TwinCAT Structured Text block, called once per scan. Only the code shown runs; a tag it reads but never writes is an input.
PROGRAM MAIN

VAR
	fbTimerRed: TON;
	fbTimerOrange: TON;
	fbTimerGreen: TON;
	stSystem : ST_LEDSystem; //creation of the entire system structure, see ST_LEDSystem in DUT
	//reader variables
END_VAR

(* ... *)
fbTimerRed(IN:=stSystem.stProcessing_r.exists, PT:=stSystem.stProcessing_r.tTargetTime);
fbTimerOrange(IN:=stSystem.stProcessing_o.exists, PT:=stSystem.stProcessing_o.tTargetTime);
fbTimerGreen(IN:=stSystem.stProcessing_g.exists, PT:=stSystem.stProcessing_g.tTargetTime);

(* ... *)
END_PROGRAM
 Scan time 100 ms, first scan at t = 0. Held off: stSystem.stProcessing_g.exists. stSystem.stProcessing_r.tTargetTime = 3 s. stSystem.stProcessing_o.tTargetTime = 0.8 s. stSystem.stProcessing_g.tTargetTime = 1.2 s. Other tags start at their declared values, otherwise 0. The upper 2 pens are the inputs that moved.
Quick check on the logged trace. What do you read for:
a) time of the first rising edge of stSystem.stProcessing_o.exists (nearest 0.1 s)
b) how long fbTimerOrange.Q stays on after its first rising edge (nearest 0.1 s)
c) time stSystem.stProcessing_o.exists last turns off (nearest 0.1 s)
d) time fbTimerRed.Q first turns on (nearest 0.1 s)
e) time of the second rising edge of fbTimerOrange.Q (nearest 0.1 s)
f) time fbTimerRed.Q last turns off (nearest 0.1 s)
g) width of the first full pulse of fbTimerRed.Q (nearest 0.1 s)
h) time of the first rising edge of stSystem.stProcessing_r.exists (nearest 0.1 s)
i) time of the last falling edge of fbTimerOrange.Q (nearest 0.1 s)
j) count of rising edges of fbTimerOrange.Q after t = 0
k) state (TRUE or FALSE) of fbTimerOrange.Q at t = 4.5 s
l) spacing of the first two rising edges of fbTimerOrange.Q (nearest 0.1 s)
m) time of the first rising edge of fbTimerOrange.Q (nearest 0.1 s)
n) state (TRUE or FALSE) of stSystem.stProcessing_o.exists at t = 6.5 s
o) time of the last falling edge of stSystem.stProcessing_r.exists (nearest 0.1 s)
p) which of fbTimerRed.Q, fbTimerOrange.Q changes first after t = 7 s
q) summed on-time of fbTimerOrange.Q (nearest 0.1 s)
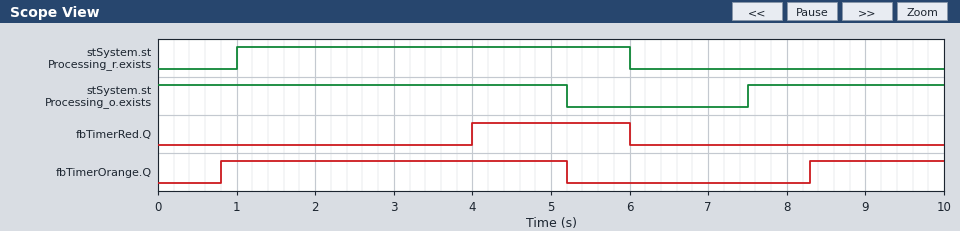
7.5 s
4.4 s
5.2 s
4.0 s
8.3 s
6.0 s
2.0 s
1.0 s
5.2 s
2
TRUE
7.5 s
0.8 s
FALSE
6.0 s
fbTimerOrange.Q
6.1 s
